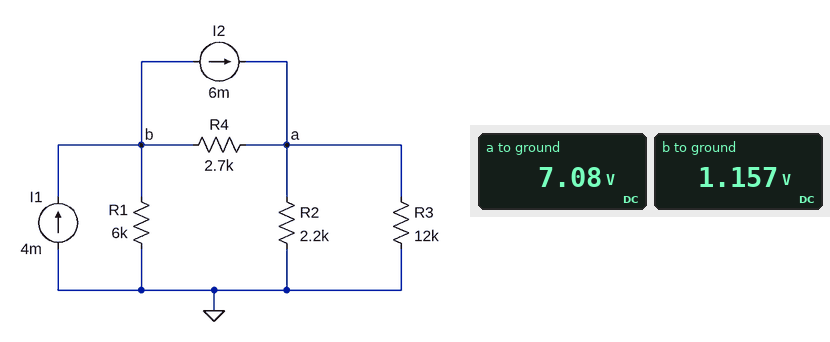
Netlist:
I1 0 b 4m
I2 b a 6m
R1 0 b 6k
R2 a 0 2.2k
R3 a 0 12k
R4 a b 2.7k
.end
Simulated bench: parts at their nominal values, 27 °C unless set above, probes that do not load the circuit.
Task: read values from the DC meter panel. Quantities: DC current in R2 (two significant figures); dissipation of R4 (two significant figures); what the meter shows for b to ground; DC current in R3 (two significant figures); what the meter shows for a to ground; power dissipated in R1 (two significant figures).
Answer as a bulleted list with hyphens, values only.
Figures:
- 3.2 mA
- 13 mW
- 1.157 V
- 590 µA
- 7.08 V
- 220 µW
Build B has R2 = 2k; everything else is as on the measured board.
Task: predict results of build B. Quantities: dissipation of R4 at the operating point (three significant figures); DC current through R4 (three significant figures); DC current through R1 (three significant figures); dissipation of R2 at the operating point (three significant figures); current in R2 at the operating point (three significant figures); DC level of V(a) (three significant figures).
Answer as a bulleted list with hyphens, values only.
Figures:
- 12.4 mW
- 2.14 mA
- 140 µA
- 21.9 mW
- 3.31 mA
- 6.62 V
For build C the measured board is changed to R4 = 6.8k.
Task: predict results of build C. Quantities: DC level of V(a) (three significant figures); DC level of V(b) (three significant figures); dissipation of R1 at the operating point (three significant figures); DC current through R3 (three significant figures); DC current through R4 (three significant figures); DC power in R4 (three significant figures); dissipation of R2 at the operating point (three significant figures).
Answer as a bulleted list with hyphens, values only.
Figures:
- 8.22 V
- -2.52 V
- 1.06 mW
- 685 µA
- 1.58 mA
- 17.0 mW
- 30.7 mW
